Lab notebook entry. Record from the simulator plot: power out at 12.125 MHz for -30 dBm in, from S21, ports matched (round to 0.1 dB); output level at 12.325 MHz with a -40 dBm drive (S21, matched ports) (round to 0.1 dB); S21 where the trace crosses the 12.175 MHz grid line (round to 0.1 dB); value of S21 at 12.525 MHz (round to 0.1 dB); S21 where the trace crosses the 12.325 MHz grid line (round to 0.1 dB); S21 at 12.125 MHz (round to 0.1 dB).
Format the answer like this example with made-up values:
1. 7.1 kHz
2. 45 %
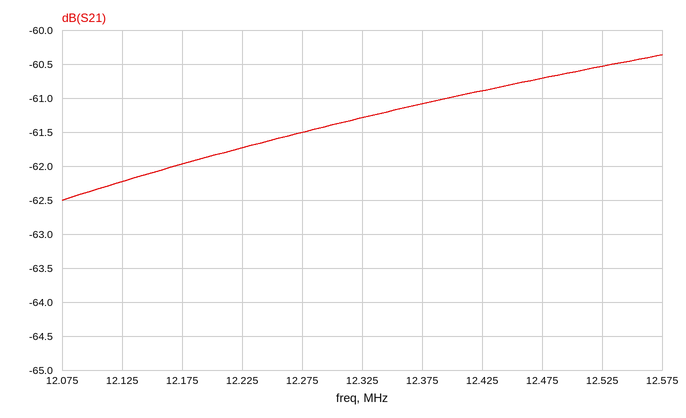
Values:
1. -92.2 dBm
2. -101.3 dBm
3. -62.0 dB
4. -60.5 dB
5. -61.3 dB
6. -62.2 dB
